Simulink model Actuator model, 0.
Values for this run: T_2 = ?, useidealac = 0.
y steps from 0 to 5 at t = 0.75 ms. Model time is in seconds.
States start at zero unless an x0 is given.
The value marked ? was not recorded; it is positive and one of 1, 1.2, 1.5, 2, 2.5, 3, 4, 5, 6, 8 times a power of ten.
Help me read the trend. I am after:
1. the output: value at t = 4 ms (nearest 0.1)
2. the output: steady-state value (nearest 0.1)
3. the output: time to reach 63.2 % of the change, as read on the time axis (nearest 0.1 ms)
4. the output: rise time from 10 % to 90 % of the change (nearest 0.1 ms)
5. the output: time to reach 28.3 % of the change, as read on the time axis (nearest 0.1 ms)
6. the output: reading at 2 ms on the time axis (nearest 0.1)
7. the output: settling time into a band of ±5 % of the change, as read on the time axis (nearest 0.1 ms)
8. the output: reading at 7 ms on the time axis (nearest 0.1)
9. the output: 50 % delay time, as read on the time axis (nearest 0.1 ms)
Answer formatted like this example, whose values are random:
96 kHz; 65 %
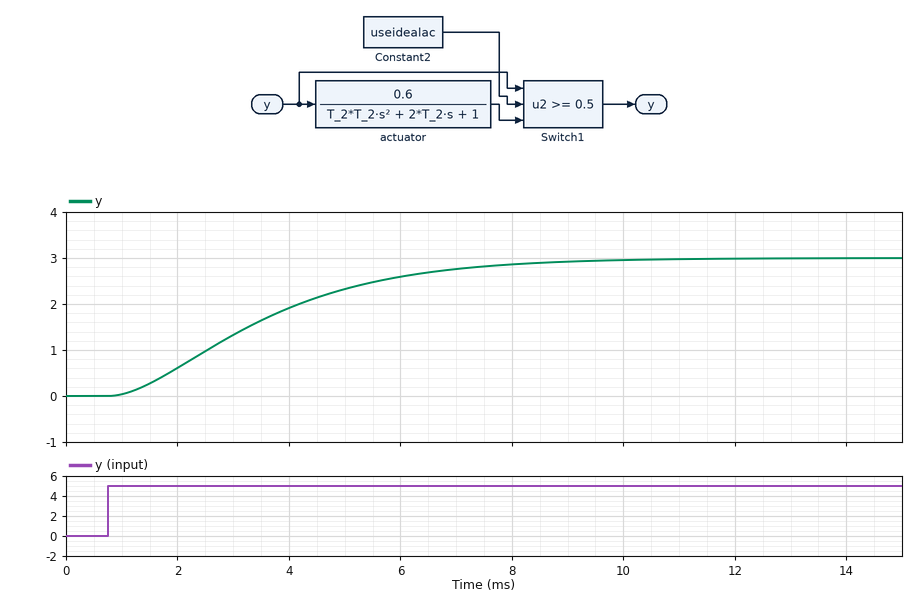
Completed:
1.9; 3.0; 4.0 ms; 5.0 ms; 2.3 ms; 0.6; 7.9 ms; 2.8; 3.3 ms
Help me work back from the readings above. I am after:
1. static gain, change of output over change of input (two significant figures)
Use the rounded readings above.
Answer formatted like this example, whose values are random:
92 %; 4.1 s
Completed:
0.60
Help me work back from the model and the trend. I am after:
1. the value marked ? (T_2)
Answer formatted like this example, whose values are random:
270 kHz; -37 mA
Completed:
0.0015
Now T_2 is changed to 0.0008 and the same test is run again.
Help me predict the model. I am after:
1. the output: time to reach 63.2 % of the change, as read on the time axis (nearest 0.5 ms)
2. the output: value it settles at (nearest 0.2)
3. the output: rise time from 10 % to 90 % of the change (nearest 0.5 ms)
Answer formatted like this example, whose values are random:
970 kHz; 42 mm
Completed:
2.5 ms; 3.0; 2.5 ms
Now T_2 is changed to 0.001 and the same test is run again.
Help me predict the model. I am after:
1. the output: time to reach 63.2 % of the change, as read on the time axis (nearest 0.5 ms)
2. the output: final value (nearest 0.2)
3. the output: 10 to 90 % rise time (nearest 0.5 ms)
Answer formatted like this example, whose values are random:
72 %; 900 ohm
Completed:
3.0 ms; 3.0; 3.5 ms
